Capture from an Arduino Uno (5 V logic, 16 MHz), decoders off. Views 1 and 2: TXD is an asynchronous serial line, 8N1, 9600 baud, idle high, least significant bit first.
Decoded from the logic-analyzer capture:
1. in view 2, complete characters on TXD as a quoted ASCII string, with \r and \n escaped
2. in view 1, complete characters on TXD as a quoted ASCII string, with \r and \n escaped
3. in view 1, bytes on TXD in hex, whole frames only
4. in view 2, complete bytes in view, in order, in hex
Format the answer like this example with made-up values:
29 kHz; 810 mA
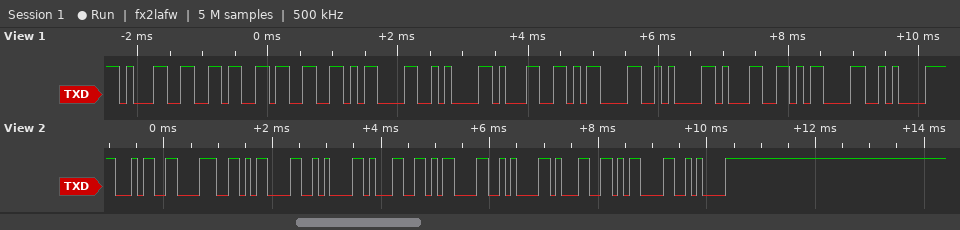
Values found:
"48\r\n1\r\n1\r\n"; "163\r\n1\r\n1\r\n"; 31 36 33 0D 0A 31 0D 0A 31 0D 0A; 34 38 0D 0A 31 0D 0A 31 0D 0A
